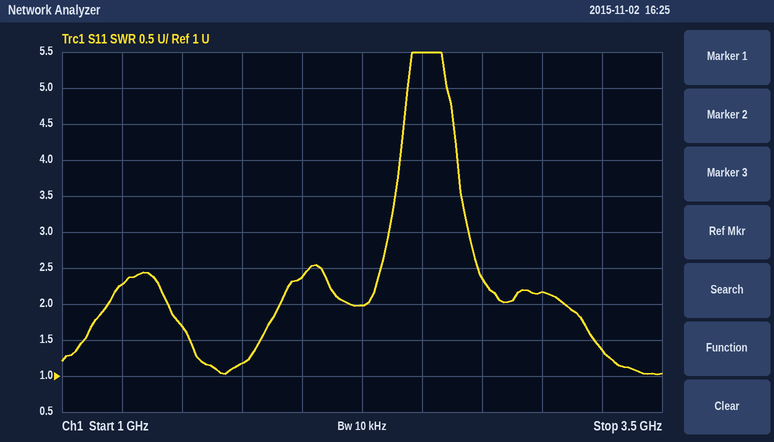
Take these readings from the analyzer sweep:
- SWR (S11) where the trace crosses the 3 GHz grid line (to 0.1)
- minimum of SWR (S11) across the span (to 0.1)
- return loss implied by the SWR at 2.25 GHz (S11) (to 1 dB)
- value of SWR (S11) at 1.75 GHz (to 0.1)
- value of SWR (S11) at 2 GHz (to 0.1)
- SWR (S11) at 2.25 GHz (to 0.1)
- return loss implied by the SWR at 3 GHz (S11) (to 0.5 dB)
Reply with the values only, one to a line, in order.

2.2
1.0
10 dB
1.2
2.4
2.0
8.5 dB
